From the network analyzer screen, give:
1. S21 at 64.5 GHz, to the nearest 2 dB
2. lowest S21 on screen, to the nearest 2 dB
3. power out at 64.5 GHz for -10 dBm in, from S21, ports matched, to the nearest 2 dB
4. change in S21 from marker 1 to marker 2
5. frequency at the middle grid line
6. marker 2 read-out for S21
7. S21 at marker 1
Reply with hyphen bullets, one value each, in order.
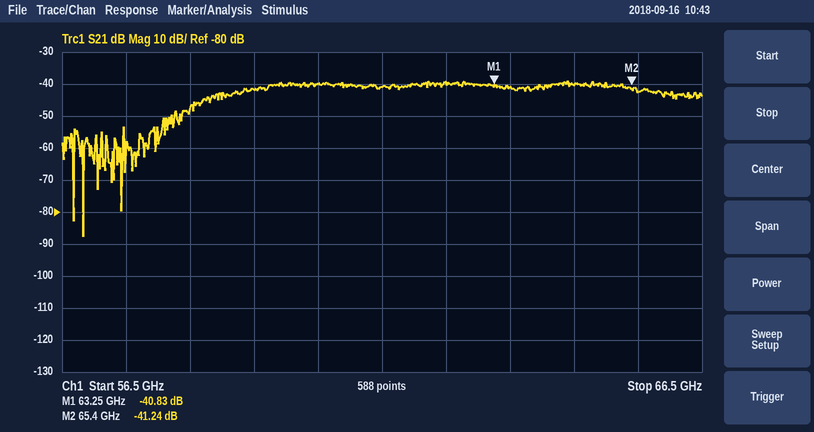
- -40 dB
- -88 dB
- -50 dBm
- -0.41 dB
- 61.5 GHz
- -41.24 dB
- -40.83 dB
